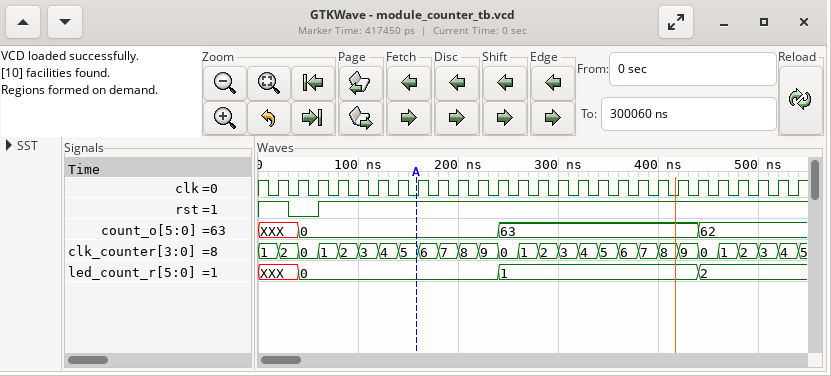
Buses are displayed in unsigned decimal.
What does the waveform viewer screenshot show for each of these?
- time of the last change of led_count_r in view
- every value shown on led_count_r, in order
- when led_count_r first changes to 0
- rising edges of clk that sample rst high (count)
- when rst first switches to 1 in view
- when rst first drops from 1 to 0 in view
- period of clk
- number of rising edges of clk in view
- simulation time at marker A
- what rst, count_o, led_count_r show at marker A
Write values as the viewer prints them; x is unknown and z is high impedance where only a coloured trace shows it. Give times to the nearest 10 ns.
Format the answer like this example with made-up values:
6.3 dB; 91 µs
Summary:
440 ns; XXX, 0, 1, 2; 40 ns; 25; 60 ns; 30 ns; 20 ns; 27; 160 ns; rst=1, count_o=0, led_count_r=0
